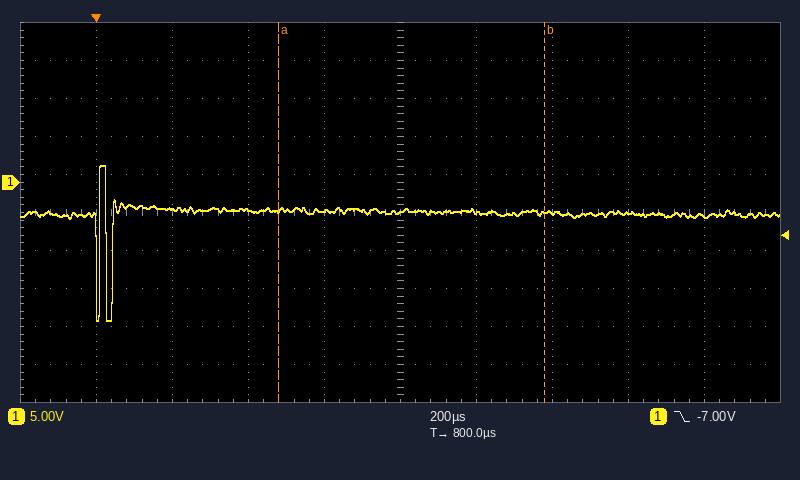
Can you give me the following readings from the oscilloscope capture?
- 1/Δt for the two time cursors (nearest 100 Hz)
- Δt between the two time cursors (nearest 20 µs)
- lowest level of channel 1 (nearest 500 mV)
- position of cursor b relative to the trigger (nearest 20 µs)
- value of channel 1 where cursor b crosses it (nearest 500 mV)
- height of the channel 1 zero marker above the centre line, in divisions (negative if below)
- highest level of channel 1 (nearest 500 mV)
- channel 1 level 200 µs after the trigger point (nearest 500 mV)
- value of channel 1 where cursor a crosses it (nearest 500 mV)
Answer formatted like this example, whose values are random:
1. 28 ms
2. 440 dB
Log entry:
1. 1.4 kHz
2. 700 µs
3. -18.0 V
4. +1.18 ms
5. -4.0 V
6. +0.8 div
7. 2.0 V
8. -3.5 V
9. -3.5 V
